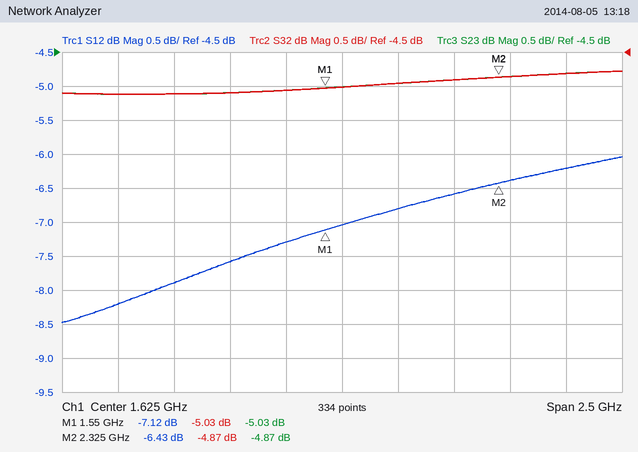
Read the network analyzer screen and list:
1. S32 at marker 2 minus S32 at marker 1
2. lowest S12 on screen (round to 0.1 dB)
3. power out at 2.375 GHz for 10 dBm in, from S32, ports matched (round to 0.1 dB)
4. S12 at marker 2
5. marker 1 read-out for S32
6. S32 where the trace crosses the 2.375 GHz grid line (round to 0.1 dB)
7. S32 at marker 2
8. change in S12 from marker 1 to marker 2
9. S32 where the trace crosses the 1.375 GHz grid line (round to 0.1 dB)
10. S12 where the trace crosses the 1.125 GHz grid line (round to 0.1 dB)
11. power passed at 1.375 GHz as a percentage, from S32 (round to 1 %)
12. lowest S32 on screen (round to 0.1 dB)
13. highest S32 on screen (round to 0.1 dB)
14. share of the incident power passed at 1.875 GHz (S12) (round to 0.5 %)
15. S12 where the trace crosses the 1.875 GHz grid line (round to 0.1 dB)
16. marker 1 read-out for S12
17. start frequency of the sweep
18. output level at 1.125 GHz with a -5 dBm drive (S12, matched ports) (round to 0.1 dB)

0.16 dB
-8.5 dB
5.1 dBm
-6.43 dB
-5.03 dB
-4.9 dB
-4.87 dB
0.69 dB
-5.1 dB
-7.6 dB
31 %
-5.1 dB
-4.8 dB
21.0 %
-6.8 dB
-7.12 dB
375 MHz
-12.6 dBm
